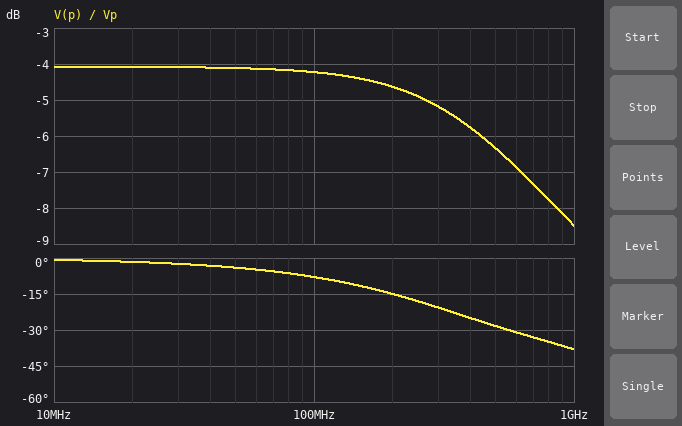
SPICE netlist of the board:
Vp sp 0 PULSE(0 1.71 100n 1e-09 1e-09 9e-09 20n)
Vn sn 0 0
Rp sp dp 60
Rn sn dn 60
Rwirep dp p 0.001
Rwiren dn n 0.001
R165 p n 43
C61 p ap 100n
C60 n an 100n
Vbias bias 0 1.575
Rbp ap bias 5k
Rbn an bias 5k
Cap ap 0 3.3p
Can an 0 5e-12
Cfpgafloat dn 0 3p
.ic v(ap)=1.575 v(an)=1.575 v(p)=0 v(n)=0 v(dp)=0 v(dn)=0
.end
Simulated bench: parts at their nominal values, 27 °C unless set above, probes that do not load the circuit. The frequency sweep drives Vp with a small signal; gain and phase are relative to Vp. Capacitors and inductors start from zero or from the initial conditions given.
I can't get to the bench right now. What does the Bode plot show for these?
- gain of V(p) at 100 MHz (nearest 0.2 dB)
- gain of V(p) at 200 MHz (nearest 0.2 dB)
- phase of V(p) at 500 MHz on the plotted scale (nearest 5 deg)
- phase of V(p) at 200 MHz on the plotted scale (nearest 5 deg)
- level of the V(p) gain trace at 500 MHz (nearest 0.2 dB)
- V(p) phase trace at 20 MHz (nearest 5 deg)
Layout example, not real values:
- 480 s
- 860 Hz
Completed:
- -4.2 dB
- -4.6 dB
- -30 deg
- -15 deg
- -6.4 dB
- 0 deg
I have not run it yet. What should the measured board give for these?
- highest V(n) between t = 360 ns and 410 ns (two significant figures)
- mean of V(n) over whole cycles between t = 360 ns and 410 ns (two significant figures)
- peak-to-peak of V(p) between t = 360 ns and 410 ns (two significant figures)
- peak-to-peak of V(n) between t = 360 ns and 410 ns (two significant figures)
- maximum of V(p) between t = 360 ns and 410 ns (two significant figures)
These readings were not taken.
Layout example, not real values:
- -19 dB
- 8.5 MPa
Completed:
- 620 mV
- 310 mV
- 1.1 V
- 620 mV
- 1.1 V
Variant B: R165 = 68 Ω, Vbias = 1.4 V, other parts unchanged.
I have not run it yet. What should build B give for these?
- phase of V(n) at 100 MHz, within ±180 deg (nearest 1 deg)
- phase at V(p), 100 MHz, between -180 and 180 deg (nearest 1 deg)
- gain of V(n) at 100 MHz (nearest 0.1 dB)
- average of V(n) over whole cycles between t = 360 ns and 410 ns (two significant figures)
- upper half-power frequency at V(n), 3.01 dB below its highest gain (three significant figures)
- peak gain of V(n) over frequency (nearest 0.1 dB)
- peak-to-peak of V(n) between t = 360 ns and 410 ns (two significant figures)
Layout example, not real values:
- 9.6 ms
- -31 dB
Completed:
- -16 deg
- -7 deg
- -10.3 dB
- 270 mV
- 412 MHz
- -10.1 dB
- 540 mV
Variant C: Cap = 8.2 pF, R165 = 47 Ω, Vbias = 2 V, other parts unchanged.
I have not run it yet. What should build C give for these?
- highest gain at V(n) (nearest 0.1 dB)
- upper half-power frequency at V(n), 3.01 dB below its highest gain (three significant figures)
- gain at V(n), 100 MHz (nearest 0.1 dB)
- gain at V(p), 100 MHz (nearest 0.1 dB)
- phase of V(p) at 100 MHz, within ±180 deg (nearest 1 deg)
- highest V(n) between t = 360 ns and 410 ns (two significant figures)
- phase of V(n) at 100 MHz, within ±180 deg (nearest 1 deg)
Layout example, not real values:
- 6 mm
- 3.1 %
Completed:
- -9.0 dB
- 309 MHz
- -9.4 dB
- -4.3 dB
- -14 deg
- 610 mV
- -22 deg
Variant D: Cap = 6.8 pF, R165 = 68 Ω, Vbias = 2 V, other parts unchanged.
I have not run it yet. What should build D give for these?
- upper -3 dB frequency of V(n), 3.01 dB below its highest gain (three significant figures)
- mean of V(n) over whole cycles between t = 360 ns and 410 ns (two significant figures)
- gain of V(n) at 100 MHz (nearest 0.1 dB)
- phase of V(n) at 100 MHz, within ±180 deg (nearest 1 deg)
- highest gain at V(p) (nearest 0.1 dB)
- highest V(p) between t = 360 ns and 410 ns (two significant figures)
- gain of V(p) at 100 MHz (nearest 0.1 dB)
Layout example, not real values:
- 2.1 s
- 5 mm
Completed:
- 325 MHz
- 270 mV
- -10.4 dB
- -21 deg
- -3.4 dB
- 1.2 V
- -3.7 dB
